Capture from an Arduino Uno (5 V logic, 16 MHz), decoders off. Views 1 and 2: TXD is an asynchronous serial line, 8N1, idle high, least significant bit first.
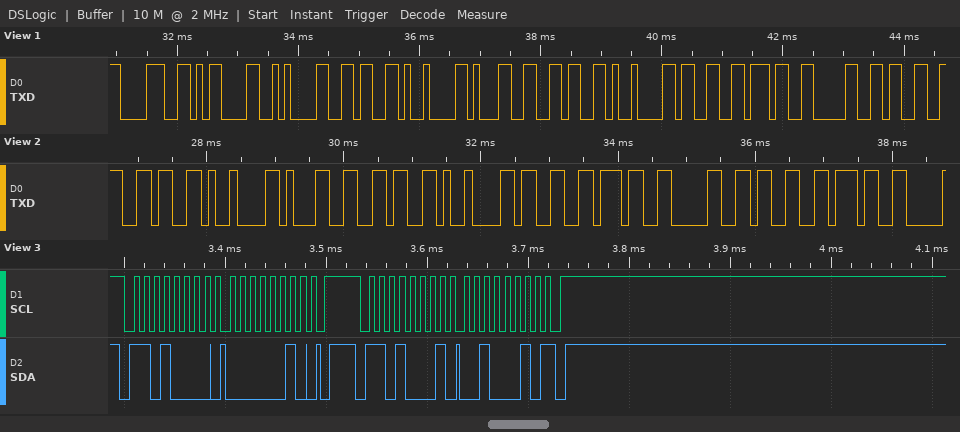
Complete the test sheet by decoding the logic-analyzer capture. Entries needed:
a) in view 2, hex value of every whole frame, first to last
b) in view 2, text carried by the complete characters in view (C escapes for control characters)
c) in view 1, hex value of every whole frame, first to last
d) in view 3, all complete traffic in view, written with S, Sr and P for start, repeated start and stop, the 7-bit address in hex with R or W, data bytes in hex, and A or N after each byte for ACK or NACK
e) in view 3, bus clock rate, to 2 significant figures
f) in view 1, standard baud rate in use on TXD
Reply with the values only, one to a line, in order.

36 09 31 36 09 33 37 30 33 37
"6\t16\t37037"
38 0D 0A 36 09 31 36 09 33 37 30 33
S 68W A 02 A P S 68R A 22 N P
100 kHz
9600 baud
